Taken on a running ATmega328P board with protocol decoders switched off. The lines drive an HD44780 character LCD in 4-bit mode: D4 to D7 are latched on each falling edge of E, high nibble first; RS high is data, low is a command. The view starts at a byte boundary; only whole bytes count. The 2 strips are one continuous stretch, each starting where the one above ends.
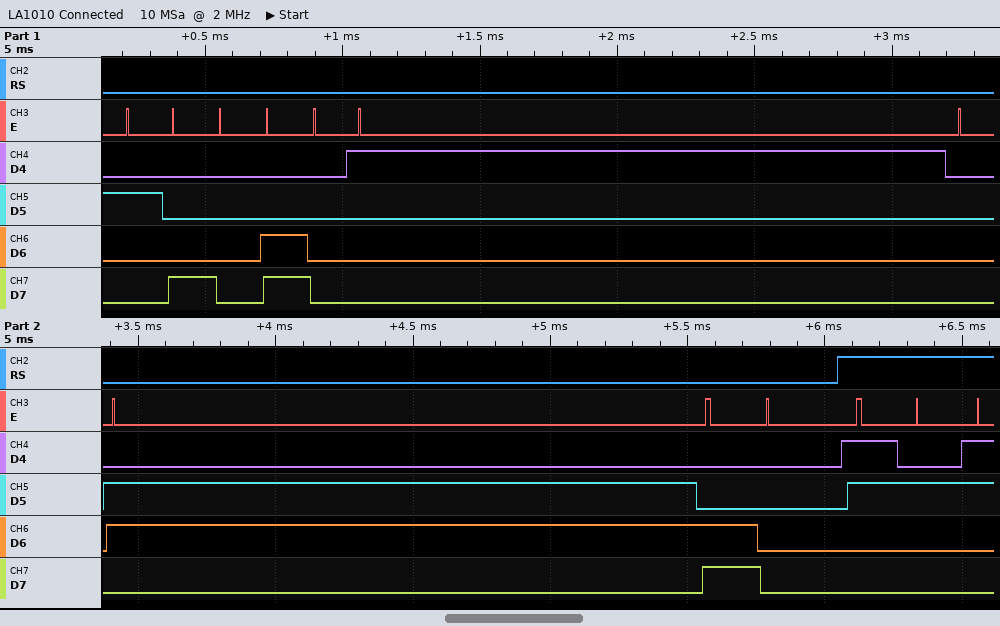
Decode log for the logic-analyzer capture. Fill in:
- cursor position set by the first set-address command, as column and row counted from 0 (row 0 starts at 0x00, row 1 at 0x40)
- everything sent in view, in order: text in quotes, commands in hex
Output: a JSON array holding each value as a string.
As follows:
["column 0, row 1", "0x28 0x0C 0x01 0x06 0xC0 \"2\""]
